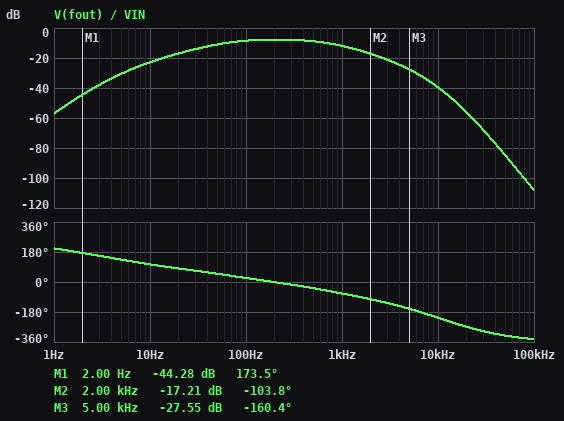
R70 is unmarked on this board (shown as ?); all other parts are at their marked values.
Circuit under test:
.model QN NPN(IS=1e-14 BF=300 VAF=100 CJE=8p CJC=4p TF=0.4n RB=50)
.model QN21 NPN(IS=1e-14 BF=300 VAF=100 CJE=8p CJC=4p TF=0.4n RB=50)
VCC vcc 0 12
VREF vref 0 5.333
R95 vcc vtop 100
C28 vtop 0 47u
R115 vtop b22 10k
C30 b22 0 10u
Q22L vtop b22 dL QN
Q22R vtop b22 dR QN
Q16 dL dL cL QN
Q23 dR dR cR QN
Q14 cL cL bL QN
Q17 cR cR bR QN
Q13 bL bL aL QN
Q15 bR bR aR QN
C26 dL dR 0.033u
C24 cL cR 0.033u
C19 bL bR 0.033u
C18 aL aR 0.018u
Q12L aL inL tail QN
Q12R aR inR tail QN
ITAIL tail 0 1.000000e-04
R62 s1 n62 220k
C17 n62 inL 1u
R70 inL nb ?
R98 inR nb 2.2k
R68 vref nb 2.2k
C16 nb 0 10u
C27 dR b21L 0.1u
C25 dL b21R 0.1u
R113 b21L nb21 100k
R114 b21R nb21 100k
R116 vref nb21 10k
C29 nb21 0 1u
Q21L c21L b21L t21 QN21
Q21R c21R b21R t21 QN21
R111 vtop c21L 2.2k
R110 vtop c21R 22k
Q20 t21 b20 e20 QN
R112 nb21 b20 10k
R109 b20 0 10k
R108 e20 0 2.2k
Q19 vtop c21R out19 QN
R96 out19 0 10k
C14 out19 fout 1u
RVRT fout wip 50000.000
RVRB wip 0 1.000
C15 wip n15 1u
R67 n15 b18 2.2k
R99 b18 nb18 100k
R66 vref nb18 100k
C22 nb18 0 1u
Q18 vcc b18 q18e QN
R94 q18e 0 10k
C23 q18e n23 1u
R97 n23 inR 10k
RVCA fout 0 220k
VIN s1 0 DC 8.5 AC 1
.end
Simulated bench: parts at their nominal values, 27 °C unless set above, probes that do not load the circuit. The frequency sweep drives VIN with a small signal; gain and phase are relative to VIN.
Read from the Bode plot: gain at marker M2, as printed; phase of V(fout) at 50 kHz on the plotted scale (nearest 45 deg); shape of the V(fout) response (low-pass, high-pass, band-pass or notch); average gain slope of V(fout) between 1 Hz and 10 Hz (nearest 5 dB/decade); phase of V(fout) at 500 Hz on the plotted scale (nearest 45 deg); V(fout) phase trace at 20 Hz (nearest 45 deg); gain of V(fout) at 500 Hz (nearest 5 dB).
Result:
-17.21 dB
-315 deg
band-pass
35 dB/decade
-45 deg
90 deg
-10 dB
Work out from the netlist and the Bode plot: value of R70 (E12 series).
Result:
1 kΩ
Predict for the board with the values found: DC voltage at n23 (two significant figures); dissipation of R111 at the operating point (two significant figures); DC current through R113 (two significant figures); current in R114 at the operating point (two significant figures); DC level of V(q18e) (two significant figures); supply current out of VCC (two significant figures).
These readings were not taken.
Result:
5.3 V
150 µW
800 nA
800 nA
4.4 V
1.6 mA
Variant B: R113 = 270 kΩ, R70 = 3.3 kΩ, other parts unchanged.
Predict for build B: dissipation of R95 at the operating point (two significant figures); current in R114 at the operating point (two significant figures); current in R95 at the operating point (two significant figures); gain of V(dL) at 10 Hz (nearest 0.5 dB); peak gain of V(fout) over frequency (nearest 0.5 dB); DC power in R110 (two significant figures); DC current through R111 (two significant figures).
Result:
95 µW
1.1 µA
970 µA
-42.0 dB
1.5 dB
2.6 mW
160 µA
